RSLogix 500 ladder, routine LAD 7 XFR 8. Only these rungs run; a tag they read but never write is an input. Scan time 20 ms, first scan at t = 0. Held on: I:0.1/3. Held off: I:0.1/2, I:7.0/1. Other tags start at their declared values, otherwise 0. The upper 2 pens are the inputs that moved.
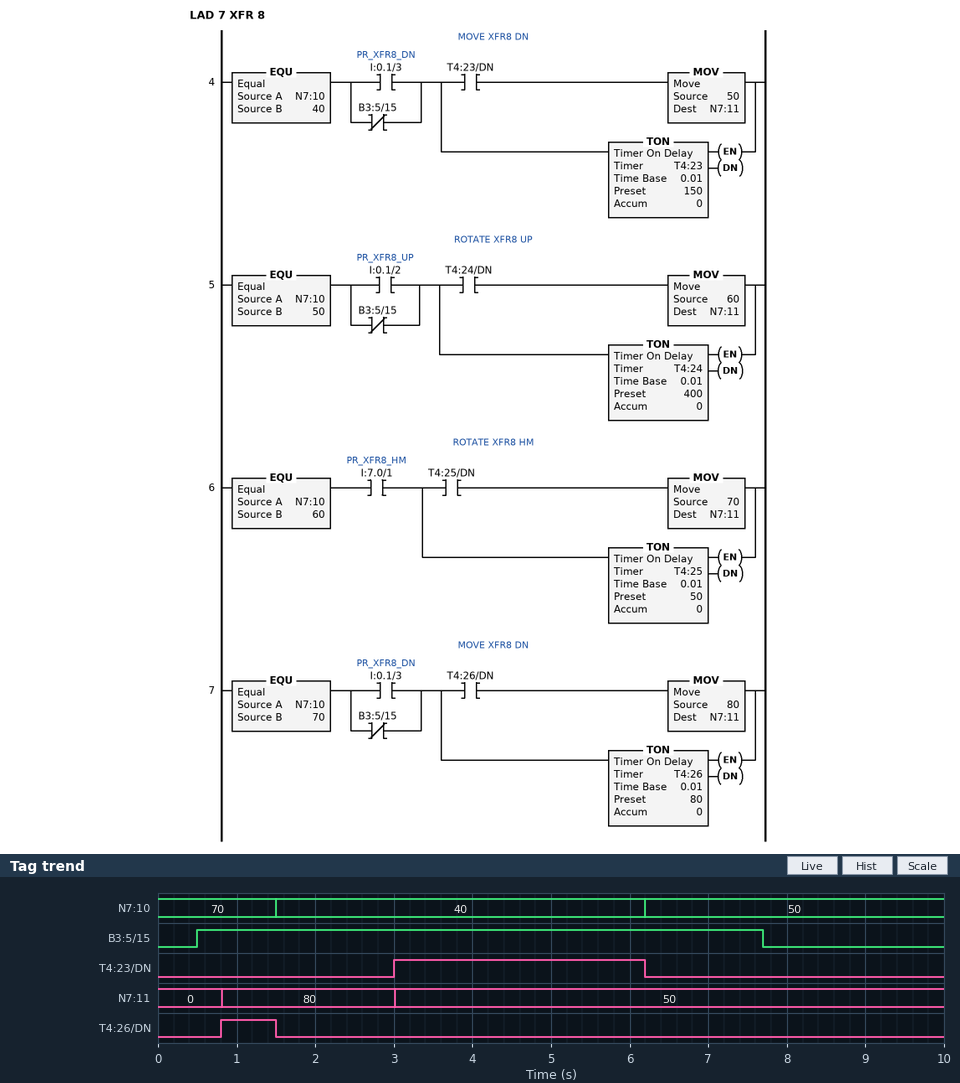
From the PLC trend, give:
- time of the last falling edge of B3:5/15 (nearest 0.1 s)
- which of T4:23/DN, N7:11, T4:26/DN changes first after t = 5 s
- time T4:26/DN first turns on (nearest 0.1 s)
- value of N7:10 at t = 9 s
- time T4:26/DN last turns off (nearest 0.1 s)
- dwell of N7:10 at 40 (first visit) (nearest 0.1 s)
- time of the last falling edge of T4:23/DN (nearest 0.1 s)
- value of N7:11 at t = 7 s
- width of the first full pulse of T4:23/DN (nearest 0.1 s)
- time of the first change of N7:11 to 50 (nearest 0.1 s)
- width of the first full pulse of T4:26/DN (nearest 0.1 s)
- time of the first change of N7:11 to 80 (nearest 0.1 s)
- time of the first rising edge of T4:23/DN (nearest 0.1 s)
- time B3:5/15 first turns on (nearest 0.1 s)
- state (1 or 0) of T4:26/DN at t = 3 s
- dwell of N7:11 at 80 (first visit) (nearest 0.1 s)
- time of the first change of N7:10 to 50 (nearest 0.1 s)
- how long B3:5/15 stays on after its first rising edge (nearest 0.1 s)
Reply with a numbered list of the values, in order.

1. 7.7 s
2. T4:23/DN
3. 0.8 s
4. 50
5. 1.5 s
6. 4.7 s
7. 6.2 s
8. 50
9. 3.2 s
10. 3.0 s
11. 0.7 s
12. 0.8 s
13. 3.0 s
14. 0.5 s
15. 0
16. 2.2 s
17. 6.2 s
18. 7.2 s
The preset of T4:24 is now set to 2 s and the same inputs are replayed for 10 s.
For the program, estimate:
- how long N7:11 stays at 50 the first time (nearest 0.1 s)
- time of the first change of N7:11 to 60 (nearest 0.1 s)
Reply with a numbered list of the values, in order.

1. 6.7 s
2. 9.7 s
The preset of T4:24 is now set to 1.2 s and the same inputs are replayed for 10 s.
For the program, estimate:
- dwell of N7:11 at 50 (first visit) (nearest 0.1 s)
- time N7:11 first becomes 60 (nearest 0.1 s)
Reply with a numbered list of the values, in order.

1. 5.9 s
2. 8.9 s
